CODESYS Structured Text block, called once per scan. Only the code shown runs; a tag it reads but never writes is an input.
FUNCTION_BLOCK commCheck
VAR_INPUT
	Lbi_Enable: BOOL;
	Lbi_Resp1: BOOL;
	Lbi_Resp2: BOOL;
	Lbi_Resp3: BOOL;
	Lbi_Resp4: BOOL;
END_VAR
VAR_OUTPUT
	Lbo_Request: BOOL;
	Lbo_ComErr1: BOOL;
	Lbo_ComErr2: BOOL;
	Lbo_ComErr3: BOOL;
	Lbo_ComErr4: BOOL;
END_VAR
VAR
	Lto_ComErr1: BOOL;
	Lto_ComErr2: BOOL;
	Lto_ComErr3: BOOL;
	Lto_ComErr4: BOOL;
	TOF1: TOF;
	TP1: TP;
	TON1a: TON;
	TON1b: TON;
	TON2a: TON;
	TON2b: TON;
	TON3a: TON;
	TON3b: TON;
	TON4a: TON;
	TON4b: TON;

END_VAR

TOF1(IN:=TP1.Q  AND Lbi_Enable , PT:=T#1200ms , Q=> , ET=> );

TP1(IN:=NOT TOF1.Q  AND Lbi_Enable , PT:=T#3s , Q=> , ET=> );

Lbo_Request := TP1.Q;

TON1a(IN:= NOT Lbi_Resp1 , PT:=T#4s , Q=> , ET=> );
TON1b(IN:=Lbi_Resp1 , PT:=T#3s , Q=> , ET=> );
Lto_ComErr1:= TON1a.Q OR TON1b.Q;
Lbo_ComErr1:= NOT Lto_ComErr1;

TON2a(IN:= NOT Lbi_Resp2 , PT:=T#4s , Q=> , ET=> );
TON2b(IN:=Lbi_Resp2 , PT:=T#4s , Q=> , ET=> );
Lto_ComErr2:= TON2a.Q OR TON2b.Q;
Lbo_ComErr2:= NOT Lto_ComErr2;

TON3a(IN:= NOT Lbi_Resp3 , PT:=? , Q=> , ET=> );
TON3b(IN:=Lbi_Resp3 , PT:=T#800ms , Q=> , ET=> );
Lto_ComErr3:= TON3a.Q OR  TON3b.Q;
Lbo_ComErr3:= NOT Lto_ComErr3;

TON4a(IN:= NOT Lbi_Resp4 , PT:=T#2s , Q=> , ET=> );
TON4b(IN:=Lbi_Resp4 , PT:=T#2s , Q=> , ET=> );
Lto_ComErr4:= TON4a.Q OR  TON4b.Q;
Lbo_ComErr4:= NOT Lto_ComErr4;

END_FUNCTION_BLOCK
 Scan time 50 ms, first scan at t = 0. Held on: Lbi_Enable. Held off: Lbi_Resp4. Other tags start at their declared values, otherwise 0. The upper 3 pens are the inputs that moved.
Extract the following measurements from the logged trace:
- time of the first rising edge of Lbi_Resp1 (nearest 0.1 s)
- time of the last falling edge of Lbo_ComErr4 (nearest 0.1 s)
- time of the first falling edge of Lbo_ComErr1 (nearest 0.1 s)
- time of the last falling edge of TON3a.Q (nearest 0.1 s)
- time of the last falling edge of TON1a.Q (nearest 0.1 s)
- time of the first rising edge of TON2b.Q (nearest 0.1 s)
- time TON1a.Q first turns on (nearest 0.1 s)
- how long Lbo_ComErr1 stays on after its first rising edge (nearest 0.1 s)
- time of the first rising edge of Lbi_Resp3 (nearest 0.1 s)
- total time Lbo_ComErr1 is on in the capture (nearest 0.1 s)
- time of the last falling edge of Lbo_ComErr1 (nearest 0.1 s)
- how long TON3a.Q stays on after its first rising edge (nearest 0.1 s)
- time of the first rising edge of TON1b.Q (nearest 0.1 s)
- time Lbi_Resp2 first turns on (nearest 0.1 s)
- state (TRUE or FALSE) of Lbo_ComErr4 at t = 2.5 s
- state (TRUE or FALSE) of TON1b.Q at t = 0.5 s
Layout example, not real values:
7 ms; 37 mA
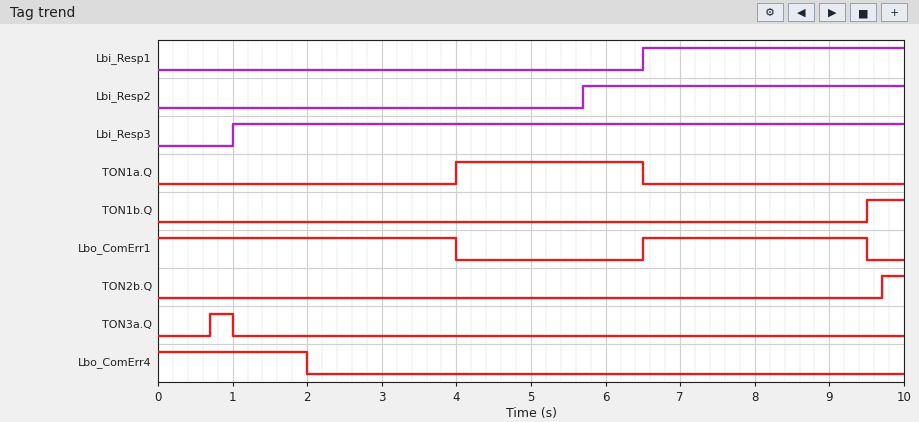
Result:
6.5 s; 2.0 s; 4.0 s; 1.0 s; 6.5 s; 9.7 s; 4.0 s; 3.0 s; 1.0 s; 7.0 s; 9.5 s; 0.3 s; 9.5 s; 5.7 s; FALSE; FALSE
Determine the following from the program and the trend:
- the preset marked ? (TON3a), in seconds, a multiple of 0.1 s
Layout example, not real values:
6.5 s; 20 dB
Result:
0.7 s
